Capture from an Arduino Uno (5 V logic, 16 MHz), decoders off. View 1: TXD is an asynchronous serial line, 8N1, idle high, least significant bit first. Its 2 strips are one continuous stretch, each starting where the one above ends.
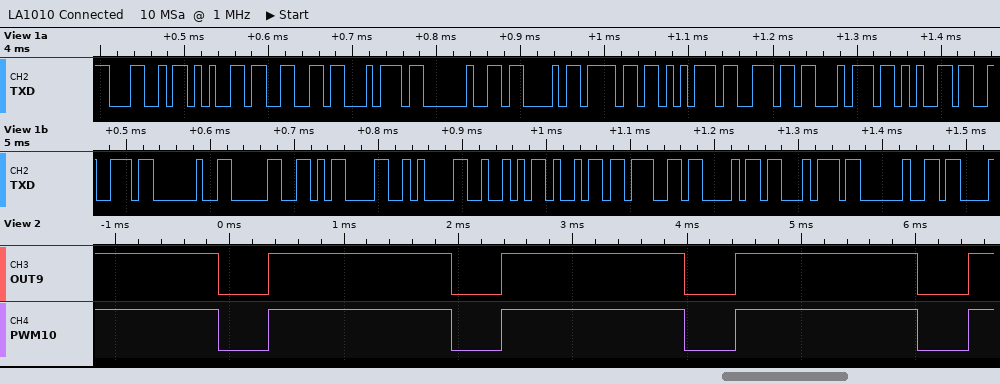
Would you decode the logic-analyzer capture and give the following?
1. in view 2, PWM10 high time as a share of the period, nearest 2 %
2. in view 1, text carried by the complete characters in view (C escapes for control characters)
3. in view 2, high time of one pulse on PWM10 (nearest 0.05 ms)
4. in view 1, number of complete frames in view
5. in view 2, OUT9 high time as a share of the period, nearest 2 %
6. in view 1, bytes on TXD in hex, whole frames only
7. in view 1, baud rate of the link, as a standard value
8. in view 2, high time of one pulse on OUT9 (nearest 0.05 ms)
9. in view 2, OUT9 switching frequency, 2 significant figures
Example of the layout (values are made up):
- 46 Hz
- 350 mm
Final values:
- 78 %
- "Left Counter 0\r\nRight "
- 1.60 ms
- 22
- 78 %
- 4C 65 66 74 20 43 6F 75 6E 74 65 72 20 30 0D 0A 52 69 67 68 74 20
- 115200 baud
- 1.60 ms
- 490 Hz
